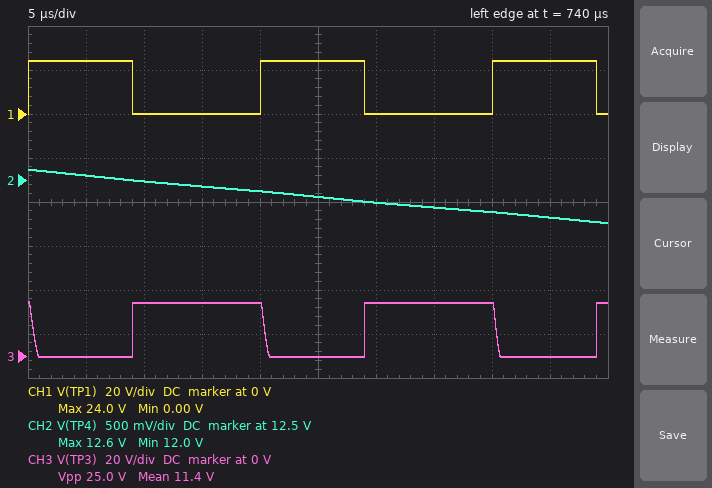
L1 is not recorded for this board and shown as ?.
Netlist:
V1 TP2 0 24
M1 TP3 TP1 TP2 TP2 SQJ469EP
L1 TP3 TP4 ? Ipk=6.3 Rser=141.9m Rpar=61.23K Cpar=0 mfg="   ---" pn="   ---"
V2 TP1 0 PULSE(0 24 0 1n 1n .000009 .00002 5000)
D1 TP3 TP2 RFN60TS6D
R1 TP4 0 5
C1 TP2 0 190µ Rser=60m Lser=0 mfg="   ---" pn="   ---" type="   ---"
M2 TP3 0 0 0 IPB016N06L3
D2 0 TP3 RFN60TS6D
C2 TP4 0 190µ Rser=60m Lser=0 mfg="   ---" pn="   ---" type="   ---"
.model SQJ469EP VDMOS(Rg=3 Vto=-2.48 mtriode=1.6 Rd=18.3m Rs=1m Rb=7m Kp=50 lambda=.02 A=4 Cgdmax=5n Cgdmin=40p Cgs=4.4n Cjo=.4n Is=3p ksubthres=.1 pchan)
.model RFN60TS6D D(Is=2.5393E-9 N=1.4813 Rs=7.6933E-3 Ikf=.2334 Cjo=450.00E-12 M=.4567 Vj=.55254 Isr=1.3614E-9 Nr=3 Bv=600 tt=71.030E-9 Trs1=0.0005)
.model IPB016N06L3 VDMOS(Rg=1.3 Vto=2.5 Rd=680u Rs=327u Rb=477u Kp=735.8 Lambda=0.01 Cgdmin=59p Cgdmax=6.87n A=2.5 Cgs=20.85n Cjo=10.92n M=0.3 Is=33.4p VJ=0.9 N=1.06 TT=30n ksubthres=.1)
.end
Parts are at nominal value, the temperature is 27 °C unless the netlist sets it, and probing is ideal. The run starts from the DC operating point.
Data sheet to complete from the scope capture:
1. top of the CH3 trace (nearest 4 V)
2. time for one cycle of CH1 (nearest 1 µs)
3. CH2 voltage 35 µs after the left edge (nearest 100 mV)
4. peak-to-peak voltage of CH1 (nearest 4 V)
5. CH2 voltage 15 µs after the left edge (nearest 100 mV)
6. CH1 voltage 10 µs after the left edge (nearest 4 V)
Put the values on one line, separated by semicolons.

24 V; 20 µs; 12.2 V; 24 V; 12.4 V; 0 V
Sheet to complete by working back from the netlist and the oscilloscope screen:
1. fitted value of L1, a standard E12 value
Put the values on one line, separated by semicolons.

680 µH
